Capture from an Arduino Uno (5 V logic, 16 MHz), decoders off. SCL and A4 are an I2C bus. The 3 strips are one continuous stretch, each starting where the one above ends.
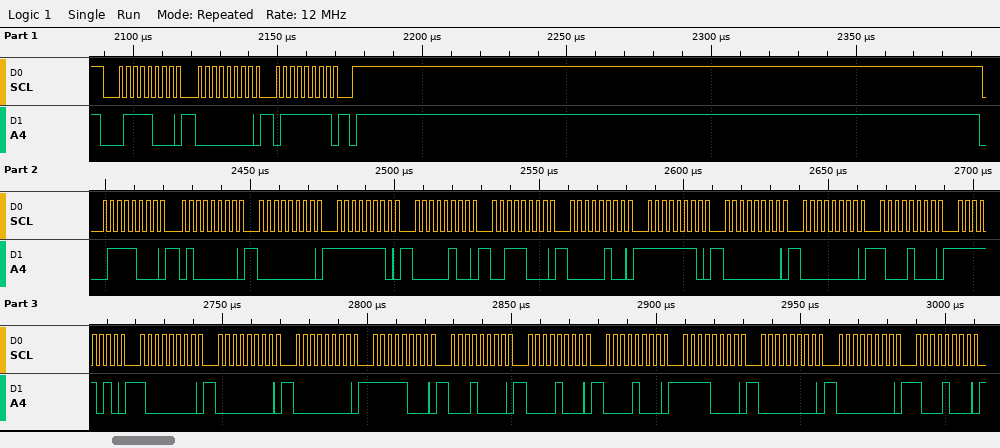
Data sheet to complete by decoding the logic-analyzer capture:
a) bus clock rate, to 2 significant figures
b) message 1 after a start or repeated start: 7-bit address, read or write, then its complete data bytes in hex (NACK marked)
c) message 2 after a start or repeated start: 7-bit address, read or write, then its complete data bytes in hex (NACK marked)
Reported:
400 kHz
0x3C write: 00 7F
0x3C write: 40 00 FE 04 38 04 FE 00 00 88 FA 80 00 00 F8 10 08 08 F0 00 00 88
